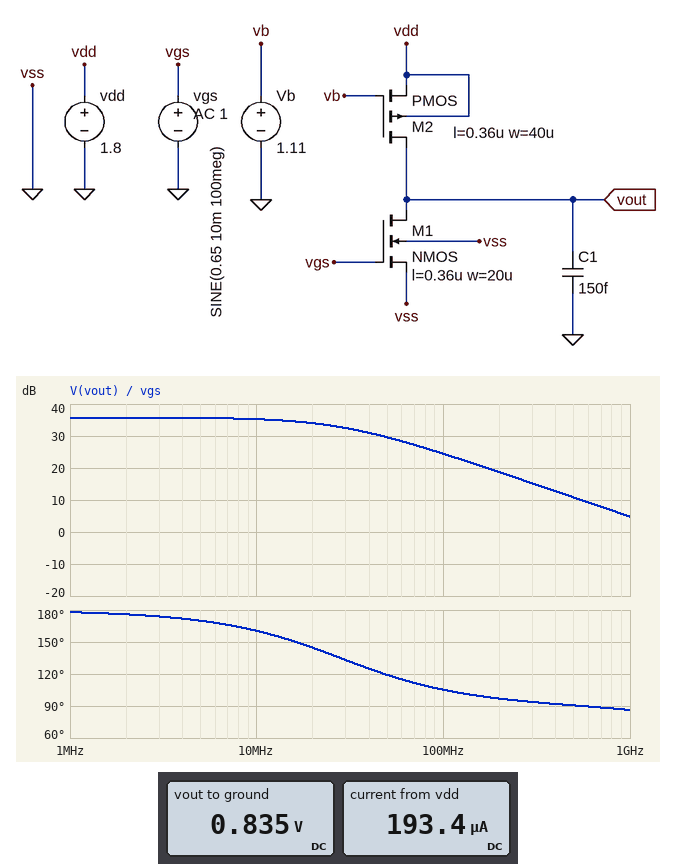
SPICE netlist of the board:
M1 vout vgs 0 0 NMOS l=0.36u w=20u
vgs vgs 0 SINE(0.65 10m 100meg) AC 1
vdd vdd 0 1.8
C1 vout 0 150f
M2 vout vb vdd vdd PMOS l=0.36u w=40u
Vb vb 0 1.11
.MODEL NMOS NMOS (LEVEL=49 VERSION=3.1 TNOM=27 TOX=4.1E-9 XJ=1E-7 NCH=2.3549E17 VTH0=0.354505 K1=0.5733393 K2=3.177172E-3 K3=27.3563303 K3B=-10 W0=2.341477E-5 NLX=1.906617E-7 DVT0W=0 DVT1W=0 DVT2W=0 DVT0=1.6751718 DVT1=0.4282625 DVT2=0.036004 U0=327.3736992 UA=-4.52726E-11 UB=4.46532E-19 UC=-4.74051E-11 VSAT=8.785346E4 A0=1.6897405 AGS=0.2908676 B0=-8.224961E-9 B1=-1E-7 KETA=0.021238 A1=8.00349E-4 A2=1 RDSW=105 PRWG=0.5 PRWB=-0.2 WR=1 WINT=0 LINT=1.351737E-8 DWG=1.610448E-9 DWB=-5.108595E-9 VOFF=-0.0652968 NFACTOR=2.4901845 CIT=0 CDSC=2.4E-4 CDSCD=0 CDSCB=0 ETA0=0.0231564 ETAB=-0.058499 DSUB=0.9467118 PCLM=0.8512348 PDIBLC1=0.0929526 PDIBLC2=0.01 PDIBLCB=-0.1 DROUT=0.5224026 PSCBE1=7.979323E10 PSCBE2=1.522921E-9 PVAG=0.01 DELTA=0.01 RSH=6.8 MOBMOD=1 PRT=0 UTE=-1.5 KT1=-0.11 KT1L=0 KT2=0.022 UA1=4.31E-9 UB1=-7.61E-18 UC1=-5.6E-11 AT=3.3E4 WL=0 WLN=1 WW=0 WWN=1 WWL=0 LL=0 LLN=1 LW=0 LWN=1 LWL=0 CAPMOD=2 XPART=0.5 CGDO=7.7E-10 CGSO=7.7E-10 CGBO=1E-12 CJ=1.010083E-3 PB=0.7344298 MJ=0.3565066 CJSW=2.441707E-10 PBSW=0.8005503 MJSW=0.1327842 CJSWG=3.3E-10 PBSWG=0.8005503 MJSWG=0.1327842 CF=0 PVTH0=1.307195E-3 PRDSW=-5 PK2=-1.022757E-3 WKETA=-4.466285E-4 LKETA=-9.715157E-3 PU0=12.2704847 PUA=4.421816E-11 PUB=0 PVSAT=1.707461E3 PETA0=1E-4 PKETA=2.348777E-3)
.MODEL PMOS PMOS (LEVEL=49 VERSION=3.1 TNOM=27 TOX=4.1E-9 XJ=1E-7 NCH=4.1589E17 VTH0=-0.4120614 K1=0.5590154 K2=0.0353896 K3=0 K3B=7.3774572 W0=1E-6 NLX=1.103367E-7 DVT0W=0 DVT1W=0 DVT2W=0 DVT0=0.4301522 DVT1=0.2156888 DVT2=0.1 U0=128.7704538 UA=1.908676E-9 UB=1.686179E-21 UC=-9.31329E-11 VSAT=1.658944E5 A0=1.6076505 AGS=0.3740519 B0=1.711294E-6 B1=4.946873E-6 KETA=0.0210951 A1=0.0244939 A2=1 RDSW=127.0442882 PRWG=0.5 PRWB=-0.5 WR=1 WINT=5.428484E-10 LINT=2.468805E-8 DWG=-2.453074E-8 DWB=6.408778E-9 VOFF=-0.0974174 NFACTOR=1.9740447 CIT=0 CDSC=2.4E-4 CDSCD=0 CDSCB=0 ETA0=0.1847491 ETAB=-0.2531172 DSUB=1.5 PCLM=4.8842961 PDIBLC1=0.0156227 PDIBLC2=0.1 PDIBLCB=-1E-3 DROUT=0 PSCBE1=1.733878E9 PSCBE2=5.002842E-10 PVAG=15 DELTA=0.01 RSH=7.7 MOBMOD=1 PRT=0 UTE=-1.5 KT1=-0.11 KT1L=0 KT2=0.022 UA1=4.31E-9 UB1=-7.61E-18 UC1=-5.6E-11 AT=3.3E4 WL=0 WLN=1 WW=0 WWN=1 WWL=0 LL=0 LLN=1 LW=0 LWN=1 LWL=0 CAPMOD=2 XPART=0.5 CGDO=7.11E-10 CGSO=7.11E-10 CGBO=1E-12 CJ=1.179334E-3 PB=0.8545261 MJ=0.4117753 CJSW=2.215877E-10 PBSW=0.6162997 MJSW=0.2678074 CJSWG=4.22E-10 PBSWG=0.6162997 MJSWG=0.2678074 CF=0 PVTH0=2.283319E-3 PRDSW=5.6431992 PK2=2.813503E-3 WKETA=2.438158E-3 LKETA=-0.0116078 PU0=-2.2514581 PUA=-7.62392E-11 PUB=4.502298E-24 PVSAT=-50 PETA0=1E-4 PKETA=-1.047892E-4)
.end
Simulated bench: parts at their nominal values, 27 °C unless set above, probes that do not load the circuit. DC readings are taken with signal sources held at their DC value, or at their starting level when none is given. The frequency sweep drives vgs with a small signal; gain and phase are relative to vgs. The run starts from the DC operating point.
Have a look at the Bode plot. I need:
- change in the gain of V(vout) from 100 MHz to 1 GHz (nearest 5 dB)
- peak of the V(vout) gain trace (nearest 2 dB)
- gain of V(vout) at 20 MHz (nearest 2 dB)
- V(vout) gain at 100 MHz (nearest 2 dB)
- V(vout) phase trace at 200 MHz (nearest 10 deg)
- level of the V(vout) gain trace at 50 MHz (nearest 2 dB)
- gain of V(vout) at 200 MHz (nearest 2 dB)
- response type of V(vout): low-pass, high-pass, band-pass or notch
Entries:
-20 dB
36 dB
34 dB
24 dB
100 deg
30 dB
18 dB
low-pass
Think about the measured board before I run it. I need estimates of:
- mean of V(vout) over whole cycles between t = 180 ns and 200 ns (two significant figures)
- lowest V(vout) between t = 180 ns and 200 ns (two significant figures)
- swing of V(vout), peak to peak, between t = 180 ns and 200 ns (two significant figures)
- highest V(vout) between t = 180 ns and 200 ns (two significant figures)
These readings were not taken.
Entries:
830 mV
660 mV
330 mV
990 mV
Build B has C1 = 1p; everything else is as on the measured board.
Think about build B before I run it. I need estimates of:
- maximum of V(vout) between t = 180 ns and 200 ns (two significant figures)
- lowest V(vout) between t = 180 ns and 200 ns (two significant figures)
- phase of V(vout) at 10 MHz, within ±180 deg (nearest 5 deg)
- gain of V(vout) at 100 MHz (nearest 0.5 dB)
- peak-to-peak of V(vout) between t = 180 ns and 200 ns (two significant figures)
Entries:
860 mV
790 mV
120 deg
11.0 dB
69 mV
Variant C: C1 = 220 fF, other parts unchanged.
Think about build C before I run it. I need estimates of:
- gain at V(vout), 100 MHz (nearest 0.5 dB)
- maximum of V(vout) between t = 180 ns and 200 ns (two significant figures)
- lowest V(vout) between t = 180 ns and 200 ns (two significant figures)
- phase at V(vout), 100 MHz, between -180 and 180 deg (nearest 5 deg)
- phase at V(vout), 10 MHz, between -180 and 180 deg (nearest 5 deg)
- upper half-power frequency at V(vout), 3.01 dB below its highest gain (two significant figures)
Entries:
22.0 dB
950 mV
700 mV
100 deg
155 deg
21 MHz
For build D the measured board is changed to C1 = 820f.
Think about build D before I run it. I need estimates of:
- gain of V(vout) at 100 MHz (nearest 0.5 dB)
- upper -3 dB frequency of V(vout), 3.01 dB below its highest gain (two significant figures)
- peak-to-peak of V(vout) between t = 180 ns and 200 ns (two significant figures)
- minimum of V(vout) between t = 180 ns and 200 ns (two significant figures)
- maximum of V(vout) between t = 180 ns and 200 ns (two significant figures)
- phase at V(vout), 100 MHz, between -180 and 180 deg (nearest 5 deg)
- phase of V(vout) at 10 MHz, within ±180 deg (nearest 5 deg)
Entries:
12.5 dB
6.8 MHz
83 mV
780 mV
870 mV
95 deg
125 deg
